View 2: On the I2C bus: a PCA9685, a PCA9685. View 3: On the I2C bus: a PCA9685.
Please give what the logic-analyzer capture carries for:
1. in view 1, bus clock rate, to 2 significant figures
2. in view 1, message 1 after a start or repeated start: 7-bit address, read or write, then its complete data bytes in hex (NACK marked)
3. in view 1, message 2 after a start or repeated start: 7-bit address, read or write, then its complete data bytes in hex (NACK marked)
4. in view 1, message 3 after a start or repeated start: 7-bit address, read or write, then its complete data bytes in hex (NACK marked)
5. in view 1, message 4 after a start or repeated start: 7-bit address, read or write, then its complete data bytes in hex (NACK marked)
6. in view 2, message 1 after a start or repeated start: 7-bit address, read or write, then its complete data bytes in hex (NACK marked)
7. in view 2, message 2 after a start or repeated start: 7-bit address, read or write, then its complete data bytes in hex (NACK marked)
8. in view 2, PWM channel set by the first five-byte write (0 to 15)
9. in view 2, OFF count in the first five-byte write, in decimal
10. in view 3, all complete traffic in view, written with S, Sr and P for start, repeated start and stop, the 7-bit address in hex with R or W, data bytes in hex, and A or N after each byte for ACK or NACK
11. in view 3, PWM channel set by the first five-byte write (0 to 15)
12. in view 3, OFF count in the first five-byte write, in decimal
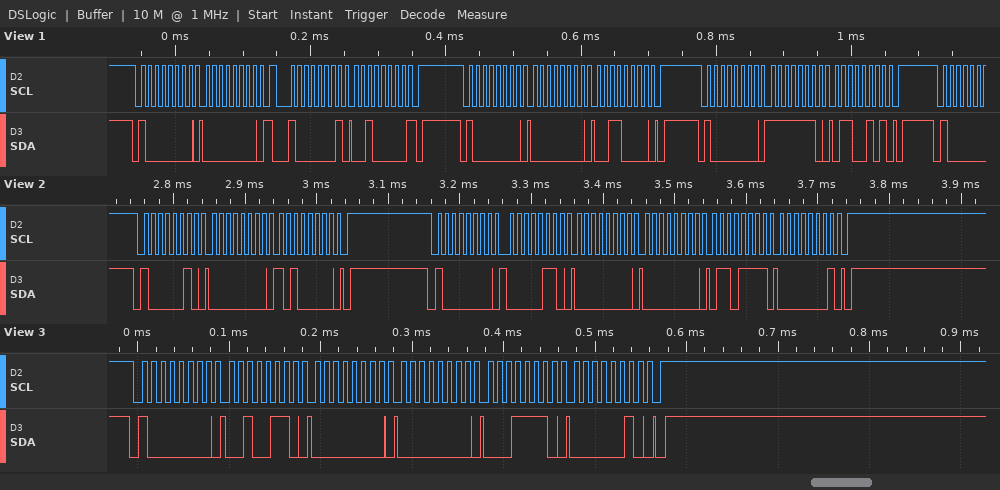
100 kHz
0x40 write: 00
0x40 read: 20 NACK
0x40 write: 00 30
0x40 write: FE 65
0x41 write: 00 A0
0x40 write: 06 00 00 6F 01
0
367
S 40W A 26 A 00 A 00 A 1E A 02 A P
8
542
